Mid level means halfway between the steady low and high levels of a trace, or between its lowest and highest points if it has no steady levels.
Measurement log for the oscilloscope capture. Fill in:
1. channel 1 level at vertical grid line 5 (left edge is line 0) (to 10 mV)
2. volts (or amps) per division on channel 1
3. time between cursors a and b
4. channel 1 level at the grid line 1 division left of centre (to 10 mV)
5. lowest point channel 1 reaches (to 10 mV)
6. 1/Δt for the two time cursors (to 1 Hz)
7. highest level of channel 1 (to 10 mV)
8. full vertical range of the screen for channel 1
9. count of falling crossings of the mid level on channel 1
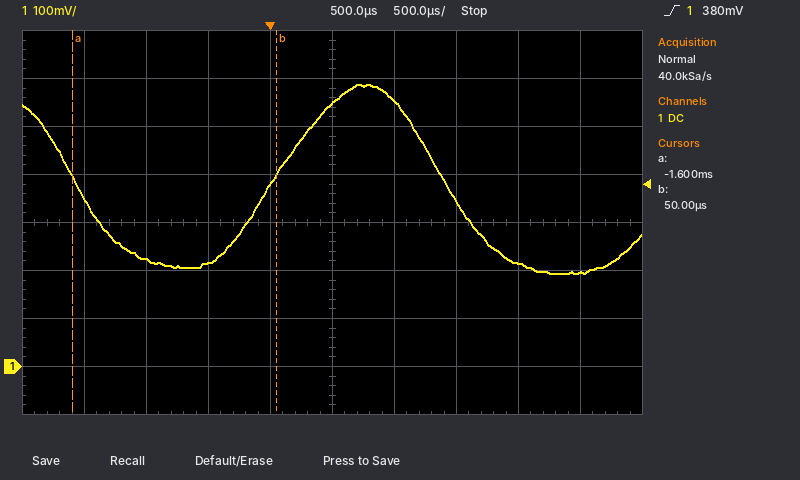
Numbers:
550 mV
100 mV
1.65 ms
380 mV
190 mV
606 Hz
590 mV
800 mV
2
